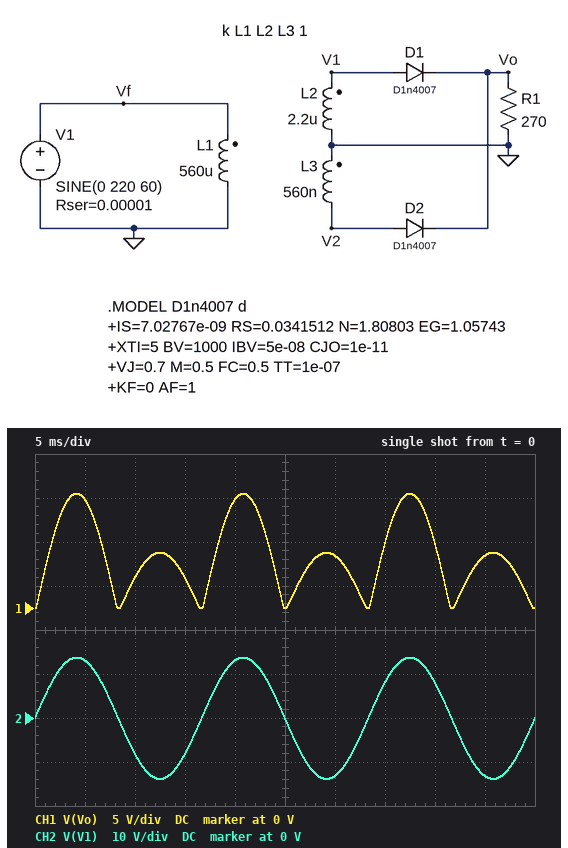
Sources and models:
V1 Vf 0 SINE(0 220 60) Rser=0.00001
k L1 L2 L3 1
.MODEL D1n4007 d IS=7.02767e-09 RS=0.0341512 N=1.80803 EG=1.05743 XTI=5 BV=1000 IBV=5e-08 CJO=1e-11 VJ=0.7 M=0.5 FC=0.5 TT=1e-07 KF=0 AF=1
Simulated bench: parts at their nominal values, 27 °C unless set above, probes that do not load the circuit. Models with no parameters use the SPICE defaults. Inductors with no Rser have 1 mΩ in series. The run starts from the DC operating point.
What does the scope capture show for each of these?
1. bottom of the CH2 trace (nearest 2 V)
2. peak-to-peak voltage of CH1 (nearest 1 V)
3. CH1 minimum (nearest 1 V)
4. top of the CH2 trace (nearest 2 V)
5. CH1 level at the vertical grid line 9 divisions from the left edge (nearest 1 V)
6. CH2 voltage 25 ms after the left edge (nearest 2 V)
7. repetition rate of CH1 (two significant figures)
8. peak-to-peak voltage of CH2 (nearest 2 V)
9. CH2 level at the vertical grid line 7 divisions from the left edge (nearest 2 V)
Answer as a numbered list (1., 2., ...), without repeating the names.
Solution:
1. -14 V
2. 13 V
3. 0 V
4. 14 V
5. 6 V
6. 0 V
7. 60 Hz
8. 28 V
9. 8 V
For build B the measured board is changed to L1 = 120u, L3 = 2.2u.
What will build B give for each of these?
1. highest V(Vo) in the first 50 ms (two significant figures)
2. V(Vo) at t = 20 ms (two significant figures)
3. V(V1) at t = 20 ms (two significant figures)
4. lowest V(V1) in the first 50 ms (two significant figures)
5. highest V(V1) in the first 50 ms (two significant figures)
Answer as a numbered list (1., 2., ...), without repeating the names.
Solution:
1. 30 V
2. 27 V
3. 28 V
4. -30 V
5. 29 V
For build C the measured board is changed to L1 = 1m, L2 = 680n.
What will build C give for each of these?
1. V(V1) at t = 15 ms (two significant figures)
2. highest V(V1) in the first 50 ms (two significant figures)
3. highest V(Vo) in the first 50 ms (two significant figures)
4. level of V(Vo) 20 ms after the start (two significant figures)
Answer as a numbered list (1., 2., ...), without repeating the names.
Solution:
1. -3.4 V
2. 5.7 V
3. 5.0 V
4. 4.8 V
